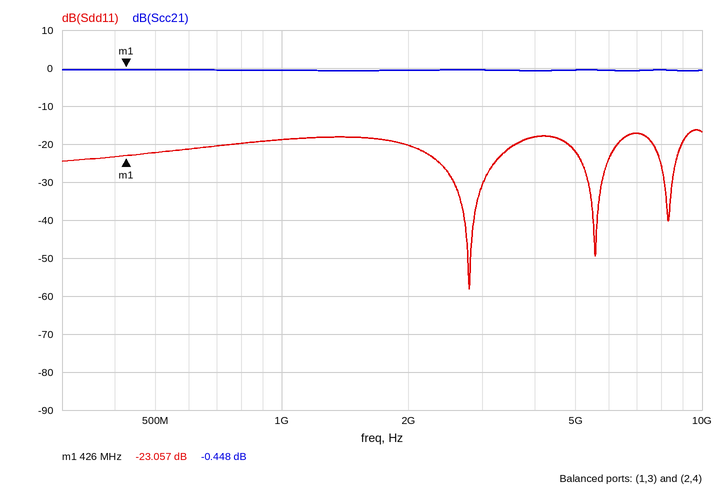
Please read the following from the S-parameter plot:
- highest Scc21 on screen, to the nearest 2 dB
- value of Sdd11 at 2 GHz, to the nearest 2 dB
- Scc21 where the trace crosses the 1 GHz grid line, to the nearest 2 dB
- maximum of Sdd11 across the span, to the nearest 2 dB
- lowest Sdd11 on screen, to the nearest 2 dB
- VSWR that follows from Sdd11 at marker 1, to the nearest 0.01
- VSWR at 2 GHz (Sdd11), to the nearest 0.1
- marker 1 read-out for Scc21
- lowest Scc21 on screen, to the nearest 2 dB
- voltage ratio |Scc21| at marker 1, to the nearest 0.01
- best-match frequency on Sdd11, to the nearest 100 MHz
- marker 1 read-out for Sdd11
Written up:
0 dB
-20 dB
0 dB
-16 dB
-58 dB
1.15
1.2
-0.448 dB
0 dB
0.95
2.8 GHz
-23.057 dB
